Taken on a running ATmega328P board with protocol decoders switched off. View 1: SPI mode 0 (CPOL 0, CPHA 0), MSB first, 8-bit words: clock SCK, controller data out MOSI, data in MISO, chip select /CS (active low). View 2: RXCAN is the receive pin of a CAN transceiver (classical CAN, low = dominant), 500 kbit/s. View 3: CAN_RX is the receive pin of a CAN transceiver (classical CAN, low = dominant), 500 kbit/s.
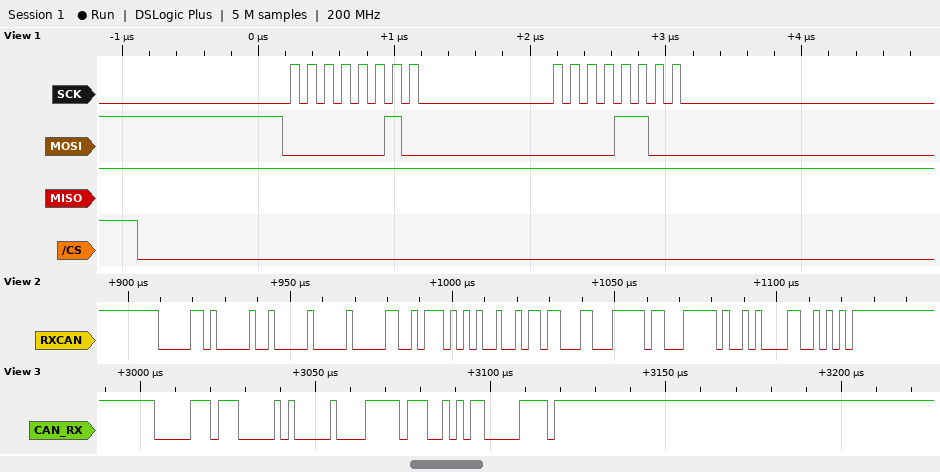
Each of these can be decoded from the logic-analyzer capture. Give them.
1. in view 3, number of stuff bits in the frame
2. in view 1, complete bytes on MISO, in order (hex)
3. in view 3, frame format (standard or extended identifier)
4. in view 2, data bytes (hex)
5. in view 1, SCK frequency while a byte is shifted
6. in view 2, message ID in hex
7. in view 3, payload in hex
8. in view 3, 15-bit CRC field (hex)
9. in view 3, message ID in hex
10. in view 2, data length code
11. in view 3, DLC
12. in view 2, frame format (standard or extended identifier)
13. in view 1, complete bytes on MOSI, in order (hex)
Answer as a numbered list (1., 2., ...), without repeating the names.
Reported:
1. 5
2. FF FF
3. standard
4. 00 09 75 49 6C 63 F8 FC
5. 8 MHz
6. 0x050
7. 00 FF
8. 0x1583
9. 0x06E
10. 8
11. 2
12. standard
13. 02 0C
